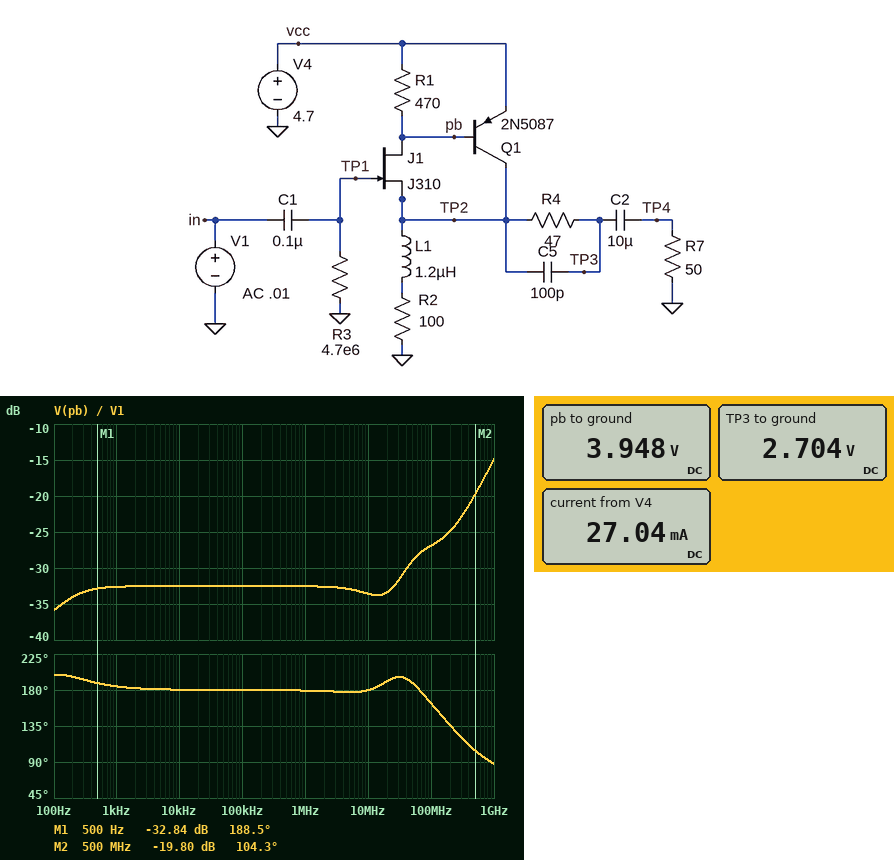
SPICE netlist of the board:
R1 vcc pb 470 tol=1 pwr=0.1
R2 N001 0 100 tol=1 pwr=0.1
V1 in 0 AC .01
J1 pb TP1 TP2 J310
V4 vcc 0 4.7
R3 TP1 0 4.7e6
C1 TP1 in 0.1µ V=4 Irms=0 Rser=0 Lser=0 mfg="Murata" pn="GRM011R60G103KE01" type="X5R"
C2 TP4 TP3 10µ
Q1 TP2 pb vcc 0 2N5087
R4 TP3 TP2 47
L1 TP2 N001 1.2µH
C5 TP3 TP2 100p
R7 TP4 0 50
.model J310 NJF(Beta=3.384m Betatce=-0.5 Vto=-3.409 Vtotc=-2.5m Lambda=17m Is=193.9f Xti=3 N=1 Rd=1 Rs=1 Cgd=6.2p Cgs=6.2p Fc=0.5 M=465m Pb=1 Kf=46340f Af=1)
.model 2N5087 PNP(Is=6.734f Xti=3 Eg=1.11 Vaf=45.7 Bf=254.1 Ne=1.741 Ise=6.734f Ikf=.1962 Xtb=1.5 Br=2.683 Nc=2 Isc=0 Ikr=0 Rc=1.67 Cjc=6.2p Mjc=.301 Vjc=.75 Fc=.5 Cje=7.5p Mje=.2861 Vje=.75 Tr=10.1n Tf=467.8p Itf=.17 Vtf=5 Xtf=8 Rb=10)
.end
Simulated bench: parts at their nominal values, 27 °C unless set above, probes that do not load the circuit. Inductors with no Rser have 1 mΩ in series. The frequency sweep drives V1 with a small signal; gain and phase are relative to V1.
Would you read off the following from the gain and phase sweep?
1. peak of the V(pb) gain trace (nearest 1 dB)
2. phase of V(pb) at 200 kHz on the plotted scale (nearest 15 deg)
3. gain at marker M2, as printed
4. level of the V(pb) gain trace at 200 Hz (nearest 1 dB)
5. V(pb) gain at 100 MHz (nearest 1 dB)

-15 dB
180 deg
-19.80 dB
-34 dB
-27 dB
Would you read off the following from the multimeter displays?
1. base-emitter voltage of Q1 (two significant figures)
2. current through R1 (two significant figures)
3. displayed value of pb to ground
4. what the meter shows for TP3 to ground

-750 mV
1.6 mA
3.948 V
2.704 V
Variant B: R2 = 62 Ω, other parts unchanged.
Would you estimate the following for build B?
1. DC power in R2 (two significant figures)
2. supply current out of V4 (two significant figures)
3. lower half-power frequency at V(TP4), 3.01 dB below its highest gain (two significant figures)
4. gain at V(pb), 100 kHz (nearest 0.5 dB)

120 mW
43 mA
160 Hz
-34.0 dB
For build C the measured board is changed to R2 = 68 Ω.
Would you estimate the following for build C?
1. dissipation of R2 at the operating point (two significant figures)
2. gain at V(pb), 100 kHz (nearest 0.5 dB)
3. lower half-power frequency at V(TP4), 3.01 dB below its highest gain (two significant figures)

110 mW
-33.5 dB
160 Hz
